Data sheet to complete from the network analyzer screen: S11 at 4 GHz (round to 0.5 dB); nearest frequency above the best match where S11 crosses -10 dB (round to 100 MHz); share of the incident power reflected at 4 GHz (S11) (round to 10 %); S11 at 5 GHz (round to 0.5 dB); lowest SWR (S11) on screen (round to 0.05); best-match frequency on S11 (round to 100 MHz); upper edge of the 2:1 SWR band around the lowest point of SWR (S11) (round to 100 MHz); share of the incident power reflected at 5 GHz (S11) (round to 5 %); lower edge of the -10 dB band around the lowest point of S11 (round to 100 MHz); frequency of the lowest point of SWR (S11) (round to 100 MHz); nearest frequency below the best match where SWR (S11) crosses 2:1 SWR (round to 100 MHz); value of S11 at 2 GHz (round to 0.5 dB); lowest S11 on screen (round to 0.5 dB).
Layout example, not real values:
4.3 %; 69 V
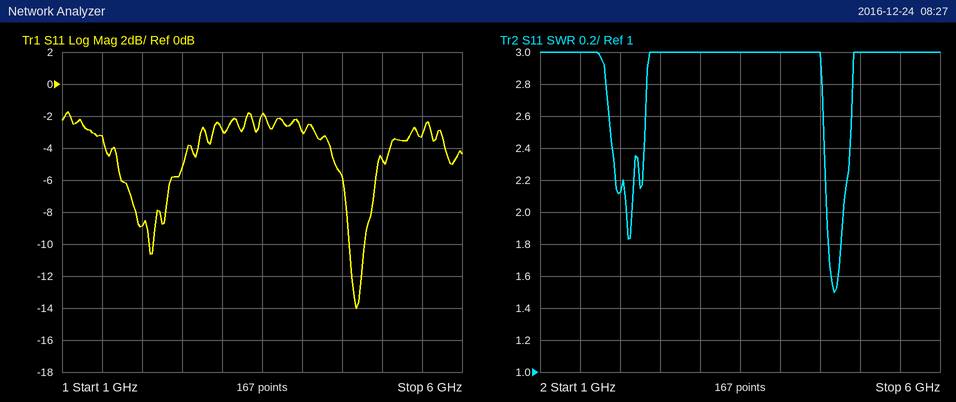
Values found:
-3.0 dB; 4.8 GHz; 50 %; -4.5 dB; 1.50; 4.7 GHz; 4.8 GHz; 35 %; 4.6 GHz; 4.7 GHz; 4.6 GHz; -9.0 dB; -14.0 dB
